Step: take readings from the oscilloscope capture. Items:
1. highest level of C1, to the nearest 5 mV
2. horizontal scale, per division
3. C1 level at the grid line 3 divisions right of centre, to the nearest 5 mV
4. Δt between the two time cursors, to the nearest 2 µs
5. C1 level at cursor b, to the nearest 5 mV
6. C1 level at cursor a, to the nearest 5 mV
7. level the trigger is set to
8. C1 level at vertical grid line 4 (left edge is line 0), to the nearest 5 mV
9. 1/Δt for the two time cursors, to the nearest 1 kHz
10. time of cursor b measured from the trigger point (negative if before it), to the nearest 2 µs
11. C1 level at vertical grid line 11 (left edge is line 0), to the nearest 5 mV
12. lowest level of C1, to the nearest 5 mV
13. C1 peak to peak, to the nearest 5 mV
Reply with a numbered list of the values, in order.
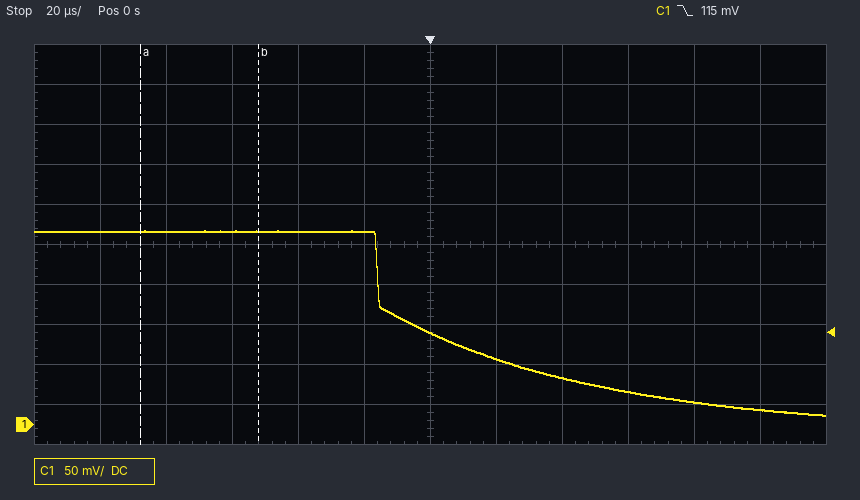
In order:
1. 240 mV
2. 20 µs
3. 40 mV
4. 36 µs
5. 240 mV
6. 240 mV
7. 115 mV
8. 240 mV
9. 28 kHz
10. -52 µs
11. 20 mV
12. 10 mV
13. 230 mV
